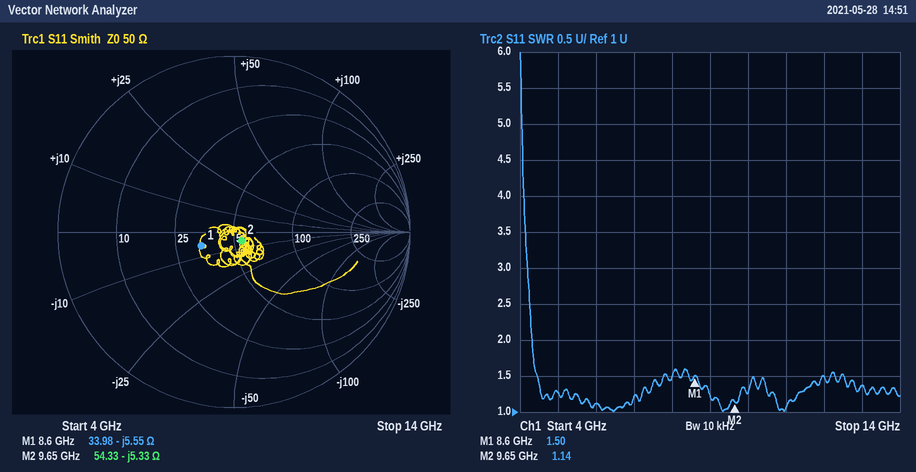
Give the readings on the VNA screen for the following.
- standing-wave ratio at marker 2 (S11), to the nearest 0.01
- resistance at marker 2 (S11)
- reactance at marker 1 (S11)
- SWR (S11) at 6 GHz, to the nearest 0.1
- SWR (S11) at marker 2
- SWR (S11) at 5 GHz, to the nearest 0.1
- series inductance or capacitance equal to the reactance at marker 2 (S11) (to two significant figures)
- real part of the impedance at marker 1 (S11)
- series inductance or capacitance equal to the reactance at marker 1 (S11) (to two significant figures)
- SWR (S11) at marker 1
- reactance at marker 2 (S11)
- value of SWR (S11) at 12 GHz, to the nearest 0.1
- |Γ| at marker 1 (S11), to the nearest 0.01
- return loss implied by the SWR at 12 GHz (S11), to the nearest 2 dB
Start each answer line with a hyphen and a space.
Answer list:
- 1.14
- 54.33 Ω
- -5.55 Ω
- 1.1
- 1.14
- 1.3
- 3.1 pF
- 33.98 Ω
- 3.3 pF
- 1.50
- -5.33 Ω
- 1.5
- 0.20
- 14 dB
